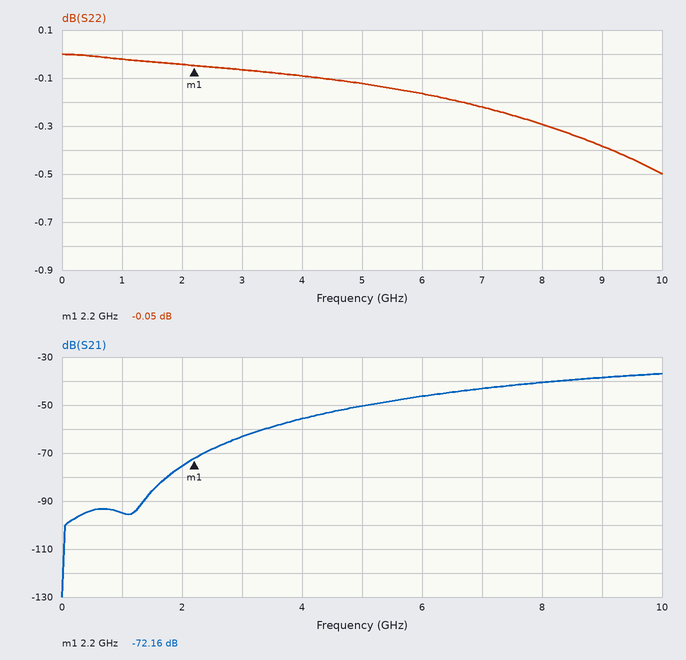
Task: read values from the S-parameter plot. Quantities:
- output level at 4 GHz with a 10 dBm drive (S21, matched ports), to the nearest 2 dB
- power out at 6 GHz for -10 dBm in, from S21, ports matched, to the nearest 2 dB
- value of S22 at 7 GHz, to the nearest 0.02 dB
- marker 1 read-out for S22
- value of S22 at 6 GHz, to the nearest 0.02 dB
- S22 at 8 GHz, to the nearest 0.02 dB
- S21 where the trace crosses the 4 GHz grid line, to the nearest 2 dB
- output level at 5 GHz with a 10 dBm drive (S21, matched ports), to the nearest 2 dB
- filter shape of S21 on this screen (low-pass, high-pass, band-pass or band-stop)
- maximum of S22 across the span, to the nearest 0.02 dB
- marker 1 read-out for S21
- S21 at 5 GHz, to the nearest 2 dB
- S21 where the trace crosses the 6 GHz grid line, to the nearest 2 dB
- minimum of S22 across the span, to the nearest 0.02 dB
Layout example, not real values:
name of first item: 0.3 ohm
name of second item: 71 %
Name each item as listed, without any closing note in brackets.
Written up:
output level at 4 GHz with a 10 dBm drive (S21, matched ports), to the nearest 2 dB: -46 dBm
power out at 6 GHz for -10 dBm in, from S21, ports matched, to the nearest 2 dB: -56 dBm
value of S22 at 7 GHz, to the nearest 0.02 dB: -0.22 dB
marker 1 read-out for S22: -0.05 dB
value of S22 at 6 GHz, to the nearest 0.02 dB: -0.16 dB
S22 at 8 GHz, to the nearest 0.02 dB: -0.30 dB
S21 where the trace crosses the 4 GHz grid line, to the nearest 2 dB: -56 dB
output level at 5 GHz with a 10 dBm drive (S21, matched ports), to the nearest 2 dB: -40 dBm
filter shape of S21 on this screen: high-pass
maximum of S22 across the span, to the nearest 0.02 dB: 0.00 dB
marker 1 read-out for S21: -72.16 dB
S21 at 5 GHz, to the nearest 2 dB: -50 dB
S21 where the trace crosses the 6 GHz grid line, to the nearest 2 dB: -46 dB
minimum of S22 across the span, to the nearest 0.02 dB: -0.50 dB
